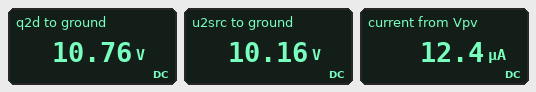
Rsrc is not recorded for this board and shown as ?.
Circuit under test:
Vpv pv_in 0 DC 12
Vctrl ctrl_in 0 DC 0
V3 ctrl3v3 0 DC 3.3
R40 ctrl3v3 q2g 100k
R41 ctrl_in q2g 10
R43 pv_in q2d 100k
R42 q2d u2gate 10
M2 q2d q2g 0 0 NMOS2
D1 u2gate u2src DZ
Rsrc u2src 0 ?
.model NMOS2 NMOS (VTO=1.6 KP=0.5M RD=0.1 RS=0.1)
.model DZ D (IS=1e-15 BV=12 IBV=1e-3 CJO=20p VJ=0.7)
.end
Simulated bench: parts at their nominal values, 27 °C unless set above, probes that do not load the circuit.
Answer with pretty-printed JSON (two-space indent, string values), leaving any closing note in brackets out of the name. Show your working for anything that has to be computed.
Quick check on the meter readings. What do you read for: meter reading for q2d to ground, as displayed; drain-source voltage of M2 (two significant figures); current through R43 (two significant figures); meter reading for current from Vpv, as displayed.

{
  "meter reading for q2d to ground, as displayed": "10.76 V",
  "drain-source voltage of M2": "10.76 V = 11 V",
  "current through R43": "(12 V - 10.76 V) / 100 kΩ = 12 µA",
  "meter reading for current from Vpv, as displayed": "12.4 µA"
}
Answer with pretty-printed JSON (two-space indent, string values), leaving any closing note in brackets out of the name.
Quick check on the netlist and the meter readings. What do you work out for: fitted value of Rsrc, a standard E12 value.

{
  "fitted value of Rsrc, a standard E12 value": "820 kΩ"
}
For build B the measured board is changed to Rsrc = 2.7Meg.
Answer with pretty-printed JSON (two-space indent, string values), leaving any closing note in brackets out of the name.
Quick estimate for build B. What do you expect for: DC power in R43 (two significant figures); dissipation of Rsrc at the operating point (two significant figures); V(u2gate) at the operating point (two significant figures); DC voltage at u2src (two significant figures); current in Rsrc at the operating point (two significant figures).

{
  "DC power in R43": "1.7 µW",
  "dissipation of Rsrc at the operating point": "45 µW",
  "V(u2gate) at the operating point": "12 V",
  "DC voltage at u2src": "11 V",
  "current in Rsrc at the operating point": "4.1 µA"
}
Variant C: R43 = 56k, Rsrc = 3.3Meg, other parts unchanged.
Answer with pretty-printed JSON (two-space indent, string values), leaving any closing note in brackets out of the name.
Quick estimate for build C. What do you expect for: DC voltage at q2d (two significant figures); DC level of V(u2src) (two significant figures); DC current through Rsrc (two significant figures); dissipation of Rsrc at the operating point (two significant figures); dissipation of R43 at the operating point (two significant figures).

{
  "DC voltage at q2d": "12 V",
  "DC level of V(u2src)": "11 V",
  "DC current through Rsrc": "3.4 µA",
  "dissipation of Rsrc at the operating point": "38 µW",
  "dissipation of R43 at the operating point": "650 nW"
}
